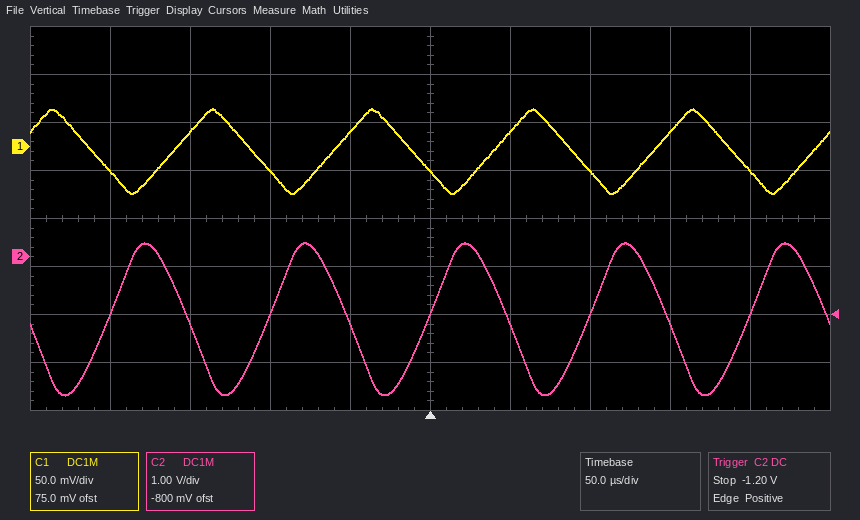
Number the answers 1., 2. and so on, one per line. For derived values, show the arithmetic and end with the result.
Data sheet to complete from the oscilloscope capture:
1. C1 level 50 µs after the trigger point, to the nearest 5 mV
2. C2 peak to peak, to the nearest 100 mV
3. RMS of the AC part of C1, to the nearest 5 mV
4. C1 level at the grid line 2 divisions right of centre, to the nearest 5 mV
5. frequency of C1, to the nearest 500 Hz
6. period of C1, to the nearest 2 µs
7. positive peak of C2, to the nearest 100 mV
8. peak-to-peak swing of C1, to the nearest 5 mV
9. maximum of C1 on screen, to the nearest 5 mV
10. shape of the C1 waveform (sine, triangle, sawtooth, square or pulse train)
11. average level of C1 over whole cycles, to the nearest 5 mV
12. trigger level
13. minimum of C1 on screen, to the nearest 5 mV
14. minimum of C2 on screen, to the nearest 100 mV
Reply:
1. 15 mV
2. 300 mV − (-2.9 V) = 3.2 V
3. 90 mV / (2√3) ≈ 26.0 mV, so 25 mV to the nearest 5 mV
4. -25 mV
5. 1 / 100 µs ≈ 10.0 kHz
6. 100 µs
7. 300 mV
8. 40 mV − (-50 mV) = 90 mV
9. 40 mV
10. triangle
11. (40 mV + (-50 mV)) / 2 ≈ -5 mV
12. -1.20 V
13. -50 mV
14. -2.9 V
